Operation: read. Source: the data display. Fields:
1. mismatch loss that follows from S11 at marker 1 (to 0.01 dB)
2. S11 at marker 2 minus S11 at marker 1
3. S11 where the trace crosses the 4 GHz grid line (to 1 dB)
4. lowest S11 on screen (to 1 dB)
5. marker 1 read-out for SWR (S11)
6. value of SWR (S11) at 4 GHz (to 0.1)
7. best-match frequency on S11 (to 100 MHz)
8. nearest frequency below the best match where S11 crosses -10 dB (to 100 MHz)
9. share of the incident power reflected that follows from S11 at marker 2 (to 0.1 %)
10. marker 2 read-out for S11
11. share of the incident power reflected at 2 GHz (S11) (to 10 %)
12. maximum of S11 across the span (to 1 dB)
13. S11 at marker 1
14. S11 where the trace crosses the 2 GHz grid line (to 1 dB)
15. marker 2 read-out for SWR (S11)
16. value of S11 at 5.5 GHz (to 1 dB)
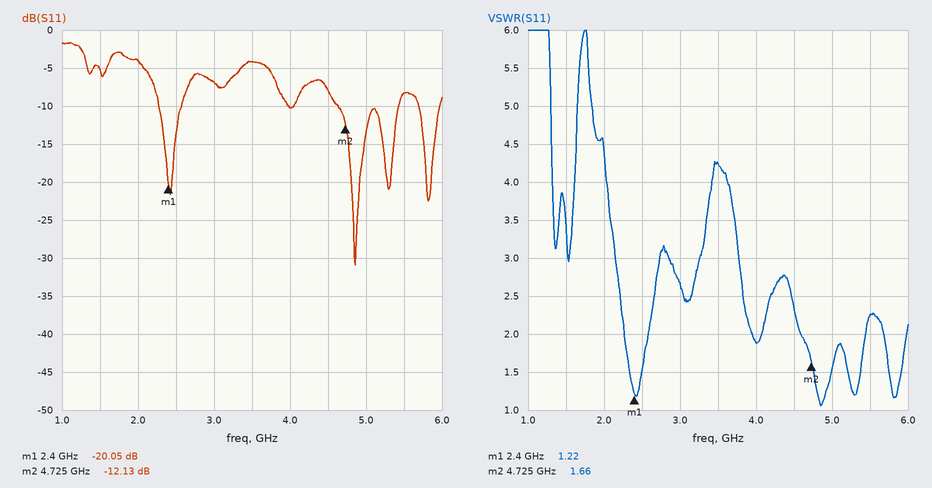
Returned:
0.04 dB
7.92 dB
-10 dB
-31 dB
1.22
1.9
4.9 GHz
4.6 GHz
6.1 %
-12.13 dB
40 %
-2 dB
-20.05 dB
-4 dB
1.66
-8 dB
